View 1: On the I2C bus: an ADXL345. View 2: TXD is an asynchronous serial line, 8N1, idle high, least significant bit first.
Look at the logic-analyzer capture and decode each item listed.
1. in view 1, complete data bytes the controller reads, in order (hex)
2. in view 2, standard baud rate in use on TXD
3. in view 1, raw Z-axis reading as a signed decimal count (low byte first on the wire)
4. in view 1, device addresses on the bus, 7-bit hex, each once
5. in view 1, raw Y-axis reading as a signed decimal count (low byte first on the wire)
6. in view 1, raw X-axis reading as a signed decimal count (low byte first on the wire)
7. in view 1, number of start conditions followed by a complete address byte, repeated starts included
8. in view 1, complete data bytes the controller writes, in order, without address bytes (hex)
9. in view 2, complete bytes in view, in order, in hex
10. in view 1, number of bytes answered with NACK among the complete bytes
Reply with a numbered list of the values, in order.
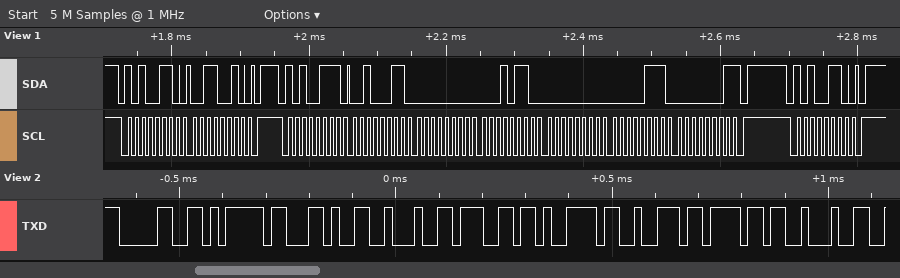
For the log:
1. 23 00 16 00 07 01
2. 57600 baud
3. 263
4. 0x53
5. 22
6. 35
7. 3
8. 32
9. 30 7D 2C 22 67 79 72 6F 22
10. 1
